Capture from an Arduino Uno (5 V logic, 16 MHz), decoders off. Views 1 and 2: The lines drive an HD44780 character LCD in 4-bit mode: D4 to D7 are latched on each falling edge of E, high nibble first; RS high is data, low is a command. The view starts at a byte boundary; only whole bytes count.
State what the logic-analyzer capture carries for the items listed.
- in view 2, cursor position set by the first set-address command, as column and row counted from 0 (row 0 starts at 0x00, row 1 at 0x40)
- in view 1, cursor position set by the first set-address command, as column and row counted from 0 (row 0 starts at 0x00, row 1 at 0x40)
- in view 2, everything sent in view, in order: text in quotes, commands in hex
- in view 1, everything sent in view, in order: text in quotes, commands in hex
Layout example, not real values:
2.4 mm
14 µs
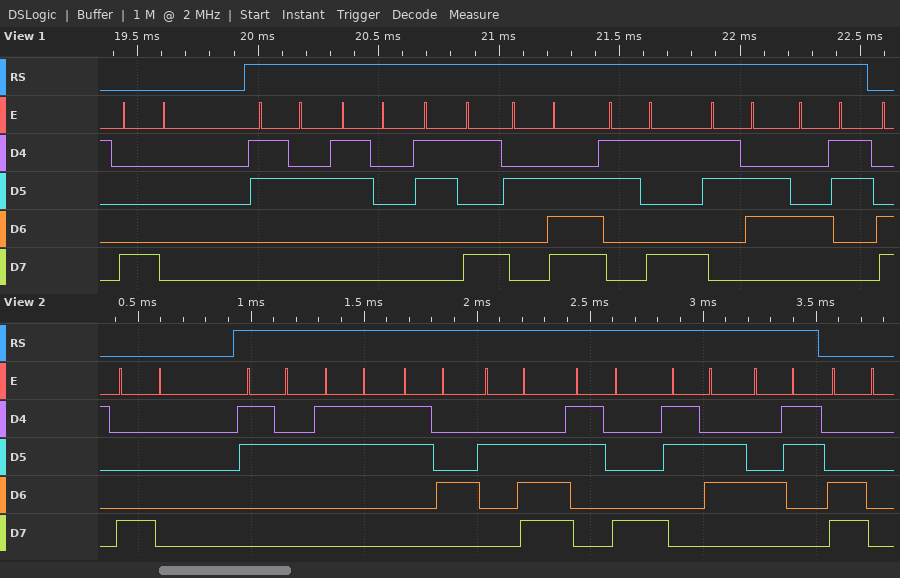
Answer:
column 0, row 0
column 0, row 0
0x80 "234.86C" 0xC0
0x80 "209.96C"
